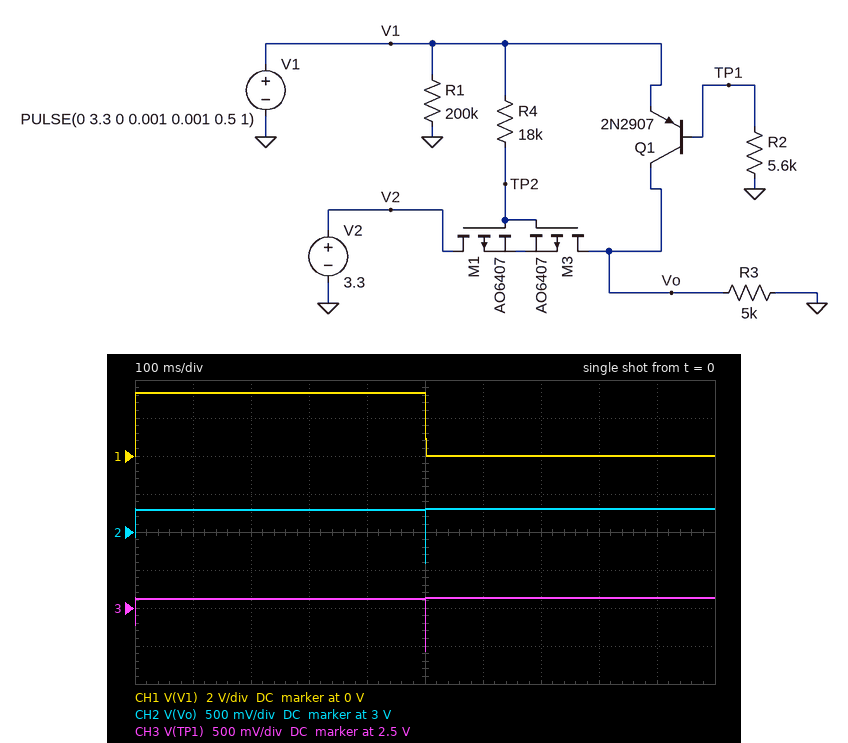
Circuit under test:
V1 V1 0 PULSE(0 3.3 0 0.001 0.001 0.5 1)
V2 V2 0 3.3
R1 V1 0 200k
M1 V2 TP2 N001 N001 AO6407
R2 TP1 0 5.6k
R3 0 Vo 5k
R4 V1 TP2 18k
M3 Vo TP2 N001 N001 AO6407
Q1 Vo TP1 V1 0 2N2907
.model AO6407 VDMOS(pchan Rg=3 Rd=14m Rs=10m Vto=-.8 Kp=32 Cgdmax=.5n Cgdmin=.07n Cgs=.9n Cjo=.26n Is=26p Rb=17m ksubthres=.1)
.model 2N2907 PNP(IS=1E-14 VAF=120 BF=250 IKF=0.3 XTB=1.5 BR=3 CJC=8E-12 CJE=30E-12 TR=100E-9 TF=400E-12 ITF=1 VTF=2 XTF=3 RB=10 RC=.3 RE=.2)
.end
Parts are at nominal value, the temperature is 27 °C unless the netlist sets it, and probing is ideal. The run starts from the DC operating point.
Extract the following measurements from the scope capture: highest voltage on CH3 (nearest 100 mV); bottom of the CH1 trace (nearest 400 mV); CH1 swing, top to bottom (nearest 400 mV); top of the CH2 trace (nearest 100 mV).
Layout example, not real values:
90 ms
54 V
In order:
2.6 V
0 V
3.2 V
3.3 V
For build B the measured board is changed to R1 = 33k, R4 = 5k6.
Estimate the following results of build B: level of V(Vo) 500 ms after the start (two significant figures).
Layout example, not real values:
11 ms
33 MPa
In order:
3.3 V
